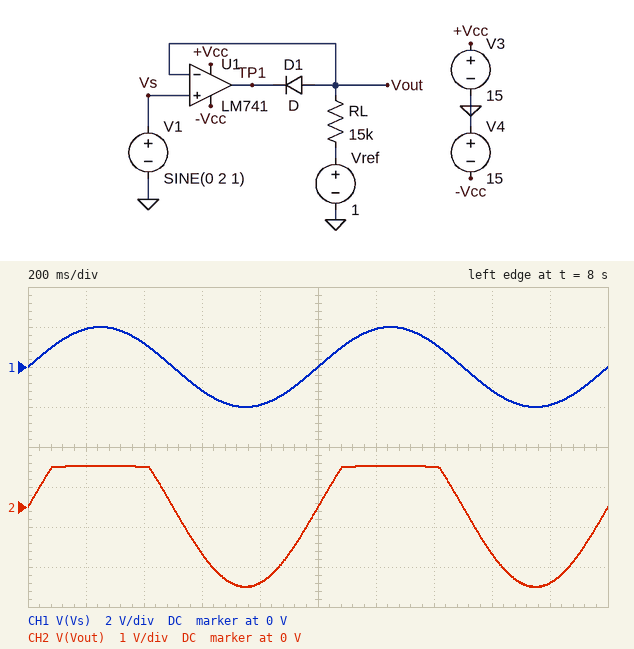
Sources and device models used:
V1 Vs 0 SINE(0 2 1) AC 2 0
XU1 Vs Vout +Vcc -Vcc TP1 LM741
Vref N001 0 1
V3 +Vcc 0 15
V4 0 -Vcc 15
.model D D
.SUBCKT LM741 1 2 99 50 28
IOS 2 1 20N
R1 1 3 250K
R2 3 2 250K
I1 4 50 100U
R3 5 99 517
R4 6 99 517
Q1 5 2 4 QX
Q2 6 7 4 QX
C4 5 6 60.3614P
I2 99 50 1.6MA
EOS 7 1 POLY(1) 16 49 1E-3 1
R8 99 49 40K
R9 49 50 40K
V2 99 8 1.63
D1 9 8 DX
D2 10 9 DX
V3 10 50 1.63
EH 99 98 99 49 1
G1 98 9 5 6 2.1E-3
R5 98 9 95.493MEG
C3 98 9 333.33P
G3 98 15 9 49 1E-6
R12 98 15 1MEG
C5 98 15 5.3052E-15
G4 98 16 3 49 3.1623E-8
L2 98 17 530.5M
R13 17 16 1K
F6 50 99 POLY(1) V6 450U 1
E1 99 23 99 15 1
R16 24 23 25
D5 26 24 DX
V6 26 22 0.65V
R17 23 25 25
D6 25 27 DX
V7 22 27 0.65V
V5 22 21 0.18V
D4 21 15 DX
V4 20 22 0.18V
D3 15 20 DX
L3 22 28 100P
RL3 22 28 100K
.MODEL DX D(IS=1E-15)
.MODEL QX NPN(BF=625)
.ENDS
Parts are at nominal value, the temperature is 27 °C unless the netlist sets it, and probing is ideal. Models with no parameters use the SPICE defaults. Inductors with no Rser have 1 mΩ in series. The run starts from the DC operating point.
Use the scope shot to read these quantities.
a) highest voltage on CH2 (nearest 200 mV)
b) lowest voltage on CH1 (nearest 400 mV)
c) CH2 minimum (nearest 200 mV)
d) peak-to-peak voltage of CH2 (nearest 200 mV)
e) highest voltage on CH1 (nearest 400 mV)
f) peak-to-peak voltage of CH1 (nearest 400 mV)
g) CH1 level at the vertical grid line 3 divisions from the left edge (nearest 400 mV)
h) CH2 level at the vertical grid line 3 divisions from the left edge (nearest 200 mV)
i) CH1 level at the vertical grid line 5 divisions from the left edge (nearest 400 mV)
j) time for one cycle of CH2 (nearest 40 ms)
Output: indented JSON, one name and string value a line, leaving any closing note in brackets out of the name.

{
  "highest voltage on CH2": "1.0 V",
  "lowest voltage on CH1": "-2.0 V",
  "CH2 minimum": "-2.0 V",
  "peak-to-peak voltage of CH2": "3.0 V",
  "highest voltage on CH1": "2.0 V",
  "peak-to-peak voltage of CH1": "4.0 V",
  "CH1 level at the vertical grid line 3 divisions from the left edge": "-1.2 V",
  "CH2 level at the vertical grid line 3 divisions from the left edge": "-1.2 V",
  "CH1 level at the vertical grid line 5 divisions from the left edge": "0 V",
  "time for one cycle of CH2": "1.00 s"
}
